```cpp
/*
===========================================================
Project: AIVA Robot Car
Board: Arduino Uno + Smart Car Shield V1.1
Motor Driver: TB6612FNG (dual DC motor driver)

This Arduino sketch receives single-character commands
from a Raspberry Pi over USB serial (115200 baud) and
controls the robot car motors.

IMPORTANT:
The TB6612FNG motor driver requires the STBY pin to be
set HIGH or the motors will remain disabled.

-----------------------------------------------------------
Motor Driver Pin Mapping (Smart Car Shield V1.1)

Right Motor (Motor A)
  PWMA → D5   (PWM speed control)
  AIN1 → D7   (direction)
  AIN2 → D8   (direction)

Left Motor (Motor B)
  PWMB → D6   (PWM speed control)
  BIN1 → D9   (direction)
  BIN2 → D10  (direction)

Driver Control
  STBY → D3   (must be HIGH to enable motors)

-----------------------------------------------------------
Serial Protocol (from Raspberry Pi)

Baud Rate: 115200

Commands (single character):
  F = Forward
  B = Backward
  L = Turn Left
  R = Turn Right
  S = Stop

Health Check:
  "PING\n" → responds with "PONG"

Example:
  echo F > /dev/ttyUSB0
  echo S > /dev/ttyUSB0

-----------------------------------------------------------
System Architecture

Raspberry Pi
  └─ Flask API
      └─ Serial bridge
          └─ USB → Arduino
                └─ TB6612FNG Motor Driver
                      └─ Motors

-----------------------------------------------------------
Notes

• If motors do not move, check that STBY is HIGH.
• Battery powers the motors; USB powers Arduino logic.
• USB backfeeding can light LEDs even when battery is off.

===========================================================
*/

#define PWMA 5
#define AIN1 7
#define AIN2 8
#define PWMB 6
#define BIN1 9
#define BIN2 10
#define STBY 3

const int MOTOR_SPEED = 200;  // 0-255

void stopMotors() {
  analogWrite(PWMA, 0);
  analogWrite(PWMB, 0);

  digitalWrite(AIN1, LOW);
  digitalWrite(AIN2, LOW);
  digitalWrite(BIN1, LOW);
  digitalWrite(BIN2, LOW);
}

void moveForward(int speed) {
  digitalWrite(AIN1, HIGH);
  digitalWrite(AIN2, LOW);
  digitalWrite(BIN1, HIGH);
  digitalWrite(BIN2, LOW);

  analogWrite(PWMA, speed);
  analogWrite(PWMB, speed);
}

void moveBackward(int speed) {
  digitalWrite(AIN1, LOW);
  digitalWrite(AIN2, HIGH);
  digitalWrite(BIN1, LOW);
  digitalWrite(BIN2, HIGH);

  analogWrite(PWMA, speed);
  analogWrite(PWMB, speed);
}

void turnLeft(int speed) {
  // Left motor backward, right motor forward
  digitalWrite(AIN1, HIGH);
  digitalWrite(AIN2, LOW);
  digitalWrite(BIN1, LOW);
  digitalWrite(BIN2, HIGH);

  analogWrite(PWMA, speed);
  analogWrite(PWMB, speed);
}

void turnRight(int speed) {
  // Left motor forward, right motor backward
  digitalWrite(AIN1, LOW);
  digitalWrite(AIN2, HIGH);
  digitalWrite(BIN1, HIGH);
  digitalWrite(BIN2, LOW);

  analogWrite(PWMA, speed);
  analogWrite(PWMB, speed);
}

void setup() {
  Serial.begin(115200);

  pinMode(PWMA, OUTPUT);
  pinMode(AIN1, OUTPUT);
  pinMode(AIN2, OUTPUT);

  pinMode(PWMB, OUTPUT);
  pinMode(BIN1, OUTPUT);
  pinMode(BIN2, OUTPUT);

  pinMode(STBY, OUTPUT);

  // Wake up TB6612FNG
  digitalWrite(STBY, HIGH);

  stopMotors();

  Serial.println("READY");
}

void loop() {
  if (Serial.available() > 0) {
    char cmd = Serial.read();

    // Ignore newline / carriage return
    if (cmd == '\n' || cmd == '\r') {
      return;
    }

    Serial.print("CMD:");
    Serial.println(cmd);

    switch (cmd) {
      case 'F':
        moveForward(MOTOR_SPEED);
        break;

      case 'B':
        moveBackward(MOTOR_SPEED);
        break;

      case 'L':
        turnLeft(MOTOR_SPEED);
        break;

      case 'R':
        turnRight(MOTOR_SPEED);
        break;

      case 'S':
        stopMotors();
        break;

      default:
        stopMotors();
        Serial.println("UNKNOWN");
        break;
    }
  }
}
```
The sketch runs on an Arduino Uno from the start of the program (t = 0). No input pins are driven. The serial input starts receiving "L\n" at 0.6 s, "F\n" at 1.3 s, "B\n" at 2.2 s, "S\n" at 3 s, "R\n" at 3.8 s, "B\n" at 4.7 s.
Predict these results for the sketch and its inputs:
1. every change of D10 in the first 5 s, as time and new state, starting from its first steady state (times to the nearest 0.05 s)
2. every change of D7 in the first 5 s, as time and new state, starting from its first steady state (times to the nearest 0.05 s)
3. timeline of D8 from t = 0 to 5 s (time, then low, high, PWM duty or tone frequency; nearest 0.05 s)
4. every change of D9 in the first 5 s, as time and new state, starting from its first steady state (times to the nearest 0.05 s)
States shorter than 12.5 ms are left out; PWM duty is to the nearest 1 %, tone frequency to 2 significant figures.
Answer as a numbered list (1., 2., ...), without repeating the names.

1. 0 s low; 0.6 s high; 1.3 s low; 2.2 s high; 3 s low; 4.7 s high
2. 0 s low; 0.6 s high; 2.2 s low
3. 0 s low; 2.2 s high; 3 s low; 3.8 s high
4. 0 s low; 1.3 s high; 2.2 s low; 3.8 s high; 4.7 s low
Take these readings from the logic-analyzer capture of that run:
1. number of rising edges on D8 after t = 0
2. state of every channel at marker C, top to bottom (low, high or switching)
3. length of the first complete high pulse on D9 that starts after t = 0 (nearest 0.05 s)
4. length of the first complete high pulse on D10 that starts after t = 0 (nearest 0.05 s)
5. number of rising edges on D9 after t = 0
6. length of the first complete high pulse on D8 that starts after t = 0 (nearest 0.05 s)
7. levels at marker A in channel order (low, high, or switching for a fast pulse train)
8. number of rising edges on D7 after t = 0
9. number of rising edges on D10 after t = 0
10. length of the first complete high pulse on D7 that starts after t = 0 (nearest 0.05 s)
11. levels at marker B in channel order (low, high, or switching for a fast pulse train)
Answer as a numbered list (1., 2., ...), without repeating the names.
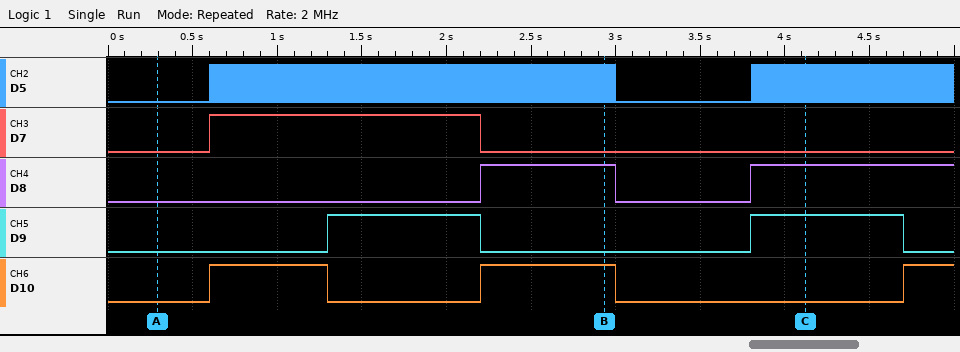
1. 2
2. D5 switching, D7 low, D8 high, D9 high, D10 low
3. 0.90 s
4. 0.70 s
5. 2
6. 0.80 s
7. D5 low, D7 low, D8 low, D9 low, D10 low
8. 1
9. 3
10. 1.60 s
11. D5 switching, D7 low, D8 high, D9 low, D10 high
